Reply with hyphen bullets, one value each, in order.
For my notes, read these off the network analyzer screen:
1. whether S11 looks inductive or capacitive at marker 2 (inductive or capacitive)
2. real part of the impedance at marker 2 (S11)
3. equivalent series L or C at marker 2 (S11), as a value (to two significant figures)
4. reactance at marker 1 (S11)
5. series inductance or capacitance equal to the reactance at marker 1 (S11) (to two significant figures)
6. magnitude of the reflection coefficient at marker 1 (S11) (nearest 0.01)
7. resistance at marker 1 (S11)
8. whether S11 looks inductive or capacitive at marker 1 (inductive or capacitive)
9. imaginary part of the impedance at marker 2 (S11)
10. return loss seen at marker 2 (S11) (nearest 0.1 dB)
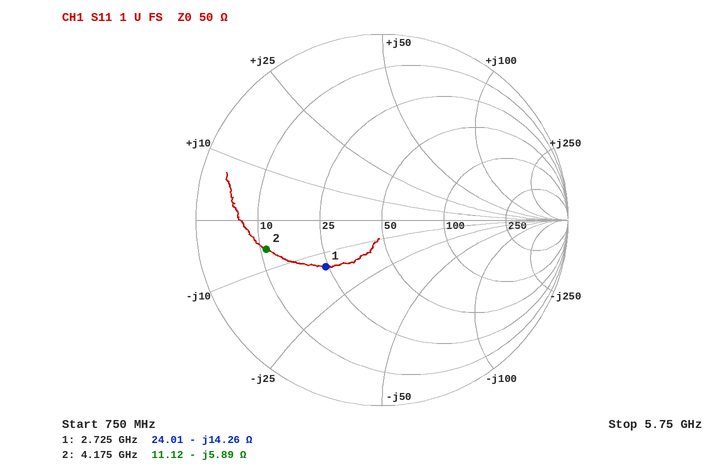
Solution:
- capacitive
- 11.12 Ω
- 6.5 pF
- -14.26 Ω
- 4.1 pF
- 0.39
- 24.01 Ω
- capacitive
- -5.89 Ω
- 3.9 dB
